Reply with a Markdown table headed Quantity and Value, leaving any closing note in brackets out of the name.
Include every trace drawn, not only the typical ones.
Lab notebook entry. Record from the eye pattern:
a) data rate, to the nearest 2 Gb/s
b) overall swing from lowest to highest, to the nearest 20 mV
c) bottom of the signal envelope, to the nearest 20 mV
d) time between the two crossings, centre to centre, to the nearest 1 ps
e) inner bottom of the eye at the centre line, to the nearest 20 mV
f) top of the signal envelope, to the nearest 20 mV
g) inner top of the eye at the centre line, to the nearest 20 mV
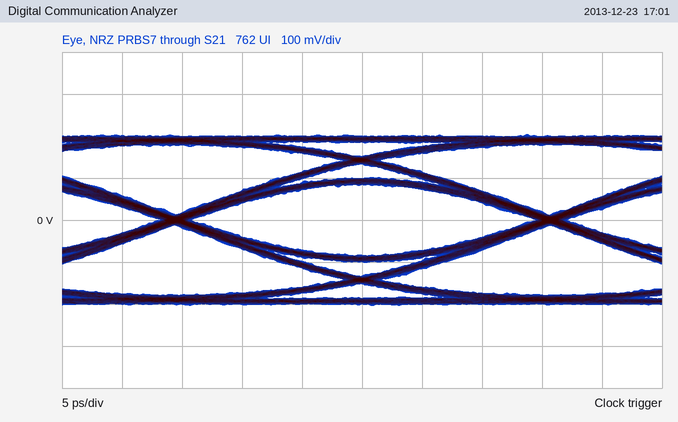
| Quantity | Value |
|---|---|
| data rate, to the nearest 2 Gb/s | 32 Gb/s |
| overall swing from lowest to highest, to the nearest 20 mV | 400 mV |
| bottom of the signal envelope, to the nearest 20 mV | -200 mV |
| time between the two crossings, centre to centre, to the nearest 1 ps | 31 ps |
| inner bottom of the eye at the centre line, to the nearest 20 mV | -80 mV |
| top of the signal envelope, to the nearest 20 mV | 200 mV |
| inner top of the eye at the centre line, to the nearest 20 mV | 80 mV |
